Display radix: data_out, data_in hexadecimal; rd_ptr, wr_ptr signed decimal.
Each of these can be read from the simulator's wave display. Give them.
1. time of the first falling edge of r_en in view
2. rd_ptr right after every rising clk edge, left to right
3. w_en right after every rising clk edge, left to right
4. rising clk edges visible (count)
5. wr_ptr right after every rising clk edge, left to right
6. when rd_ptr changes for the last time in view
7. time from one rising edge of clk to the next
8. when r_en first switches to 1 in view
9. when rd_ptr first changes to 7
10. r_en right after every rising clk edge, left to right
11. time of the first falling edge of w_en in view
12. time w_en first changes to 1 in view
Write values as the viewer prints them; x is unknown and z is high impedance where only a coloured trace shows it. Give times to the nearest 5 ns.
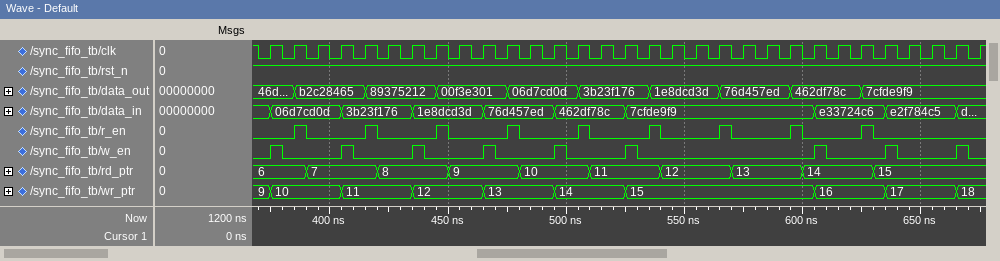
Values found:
390 ns
6, 6, 7, 7, 7, 8, 8, 8, 9, 9, 9, 10, 10, 10, 11, 11, 11, 12, 12, 12, 13, 13, 13, 14, 14, 14, 15, 15, 15, 15, 15
1 0 0 1 0 0 1 0 0 1 0 0 1 0 0 1 0 0 0 0 0 0 0 1 0 0 1 0 0 1 0
31
10, 10, 10, 11, 11, 11, 12, 12, 12, 13, 13, 13, 14, 14, 14, 15, 15, 15, 15, 15, 15, 15, 15, 16, 16, 16, 17, 17, 17, 18, 18
630 ns
10 ns
385 ns
390 ns
0 1 0 0 1 0 0 1 0 0 1 0 0 1 0 0 1 0 0 1 0 0 1 0 0 1 0 0 0 0 0
380 ns
375 ns
